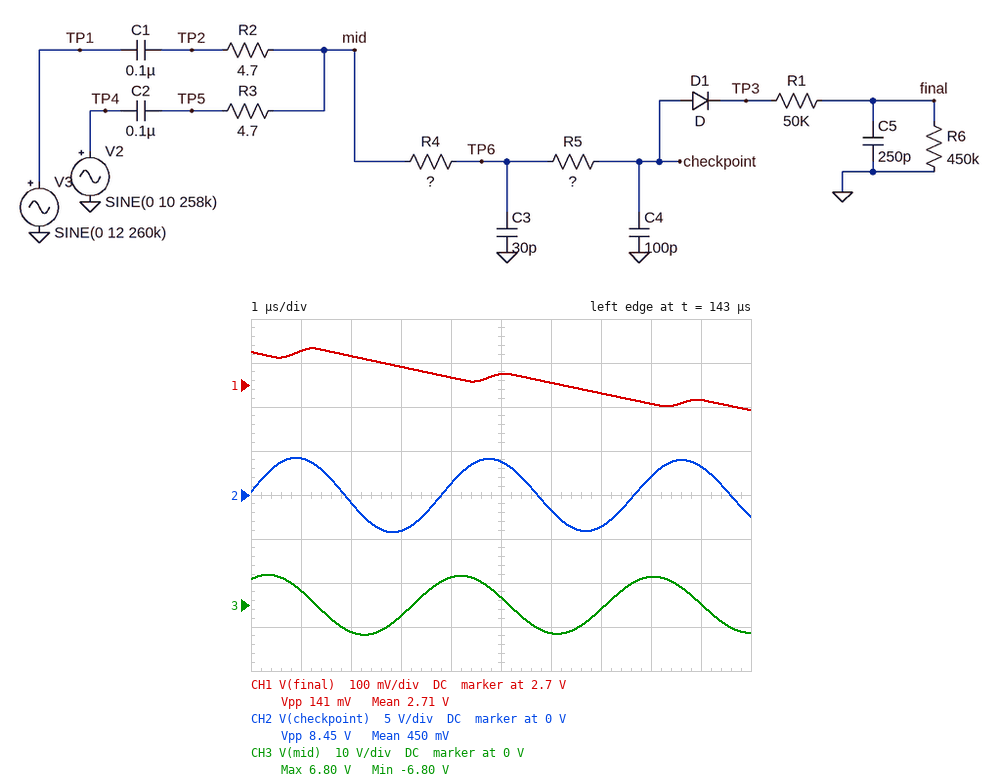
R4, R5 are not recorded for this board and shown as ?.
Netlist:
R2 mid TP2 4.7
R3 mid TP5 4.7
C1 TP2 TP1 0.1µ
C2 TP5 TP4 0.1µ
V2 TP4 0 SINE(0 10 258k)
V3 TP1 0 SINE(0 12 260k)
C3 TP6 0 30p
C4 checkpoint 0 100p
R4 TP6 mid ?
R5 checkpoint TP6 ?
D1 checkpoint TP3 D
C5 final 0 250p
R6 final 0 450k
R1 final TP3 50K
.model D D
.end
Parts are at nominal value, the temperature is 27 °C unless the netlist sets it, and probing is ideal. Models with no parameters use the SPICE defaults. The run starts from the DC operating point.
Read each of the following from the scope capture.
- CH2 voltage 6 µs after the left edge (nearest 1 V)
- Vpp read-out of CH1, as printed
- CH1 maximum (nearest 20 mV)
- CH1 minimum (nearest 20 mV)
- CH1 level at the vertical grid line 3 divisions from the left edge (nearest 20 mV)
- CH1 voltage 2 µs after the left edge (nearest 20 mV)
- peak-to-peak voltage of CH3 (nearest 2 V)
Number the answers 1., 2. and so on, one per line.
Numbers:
1. -2 V
2. 141 mV
3. 2.78 V
4. 2.64 V
5. 2.74 V
6. 2.76 V
7. 14 V
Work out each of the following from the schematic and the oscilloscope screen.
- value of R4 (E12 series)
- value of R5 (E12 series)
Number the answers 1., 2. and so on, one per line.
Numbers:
1. 820 Ω
2. 6.8 kΩ
